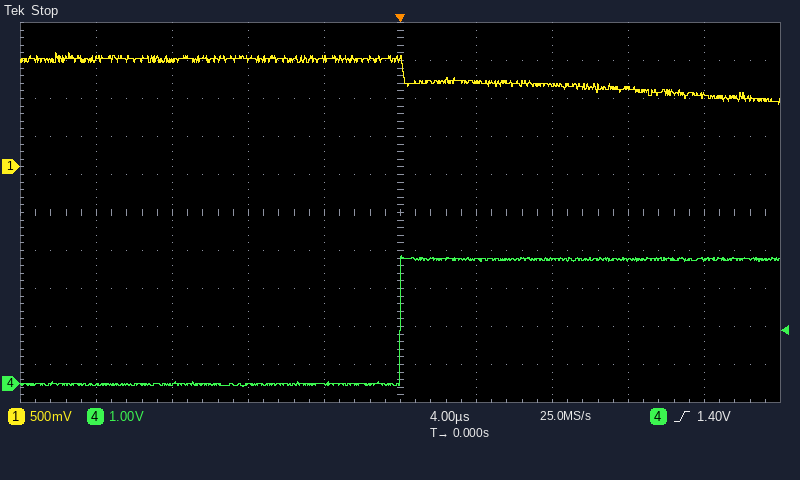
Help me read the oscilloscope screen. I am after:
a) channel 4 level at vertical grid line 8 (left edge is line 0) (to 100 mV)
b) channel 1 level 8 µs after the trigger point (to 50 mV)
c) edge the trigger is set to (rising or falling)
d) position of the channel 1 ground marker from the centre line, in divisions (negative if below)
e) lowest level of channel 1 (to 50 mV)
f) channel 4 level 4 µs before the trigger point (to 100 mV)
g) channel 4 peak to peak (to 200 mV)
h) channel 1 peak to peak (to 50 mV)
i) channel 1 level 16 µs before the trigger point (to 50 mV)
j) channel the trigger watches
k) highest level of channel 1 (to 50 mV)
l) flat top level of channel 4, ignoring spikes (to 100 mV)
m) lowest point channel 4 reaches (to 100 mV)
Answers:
3.2 V
1.10 V
rising
+1.2 div
800 mV
0.0 V
3.4 V
700 mV
1.40 V
channel 4
1.50 V
3.3 V
-100 mV
